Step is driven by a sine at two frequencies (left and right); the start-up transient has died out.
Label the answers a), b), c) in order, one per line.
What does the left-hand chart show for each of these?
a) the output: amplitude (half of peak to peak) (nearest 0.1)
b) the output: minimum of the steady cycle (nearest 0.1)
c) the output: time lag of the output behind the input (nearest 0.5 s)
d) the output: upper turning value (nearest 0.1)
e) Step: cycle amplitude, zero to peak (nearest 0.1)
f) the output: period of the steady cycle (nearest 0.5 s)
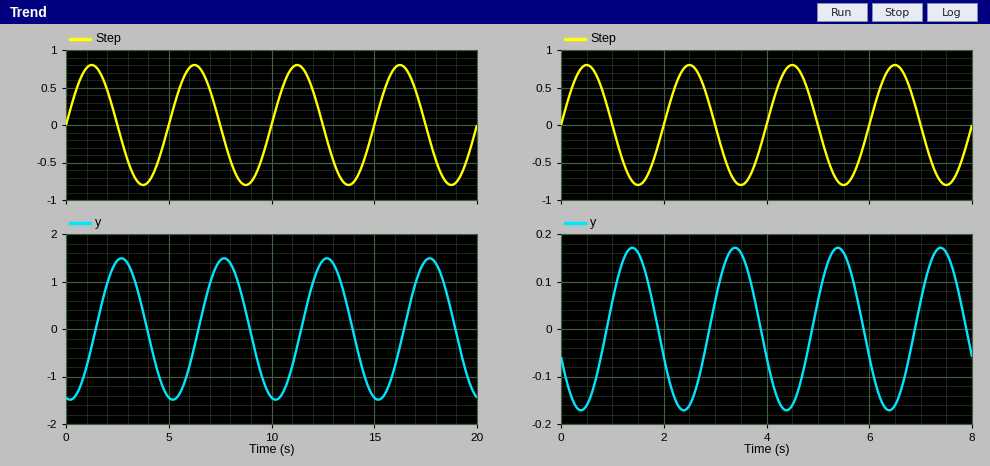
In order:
a) 1.5
b) -1.5
c) 1.5 s
d) 1.5
e) 0.8
f) 5.0 s
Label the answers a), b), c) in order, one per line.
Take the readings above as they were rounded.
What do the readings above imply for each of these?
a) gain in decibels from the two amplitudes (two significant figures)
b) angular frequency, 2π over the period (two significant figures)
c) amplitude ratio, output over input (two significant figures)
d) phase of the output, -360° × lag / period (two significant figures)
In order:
a) 5.5 dB
b) 1.3 rad/s
c) 1.9
d) -110°
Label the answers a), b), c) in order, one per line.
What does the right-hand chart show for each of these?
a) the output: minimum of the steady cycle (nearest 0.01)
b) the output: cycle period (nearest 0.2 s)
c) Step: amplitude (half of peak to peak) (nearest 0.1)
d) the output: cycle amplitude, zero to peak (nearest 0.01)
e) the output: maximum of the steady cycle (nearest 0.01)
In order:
a) -0.17
b) 2.0 s
c) 0.8
d) 0.17
e) 0.17
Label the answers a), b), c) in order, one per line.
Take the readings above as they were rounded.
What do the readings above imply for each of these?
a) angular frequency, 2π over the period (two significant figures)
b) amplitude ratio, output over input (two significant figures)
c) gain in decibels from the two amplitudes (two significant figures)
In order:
a) 3.1 rad/s
b) 0.21
c) -13 dB
